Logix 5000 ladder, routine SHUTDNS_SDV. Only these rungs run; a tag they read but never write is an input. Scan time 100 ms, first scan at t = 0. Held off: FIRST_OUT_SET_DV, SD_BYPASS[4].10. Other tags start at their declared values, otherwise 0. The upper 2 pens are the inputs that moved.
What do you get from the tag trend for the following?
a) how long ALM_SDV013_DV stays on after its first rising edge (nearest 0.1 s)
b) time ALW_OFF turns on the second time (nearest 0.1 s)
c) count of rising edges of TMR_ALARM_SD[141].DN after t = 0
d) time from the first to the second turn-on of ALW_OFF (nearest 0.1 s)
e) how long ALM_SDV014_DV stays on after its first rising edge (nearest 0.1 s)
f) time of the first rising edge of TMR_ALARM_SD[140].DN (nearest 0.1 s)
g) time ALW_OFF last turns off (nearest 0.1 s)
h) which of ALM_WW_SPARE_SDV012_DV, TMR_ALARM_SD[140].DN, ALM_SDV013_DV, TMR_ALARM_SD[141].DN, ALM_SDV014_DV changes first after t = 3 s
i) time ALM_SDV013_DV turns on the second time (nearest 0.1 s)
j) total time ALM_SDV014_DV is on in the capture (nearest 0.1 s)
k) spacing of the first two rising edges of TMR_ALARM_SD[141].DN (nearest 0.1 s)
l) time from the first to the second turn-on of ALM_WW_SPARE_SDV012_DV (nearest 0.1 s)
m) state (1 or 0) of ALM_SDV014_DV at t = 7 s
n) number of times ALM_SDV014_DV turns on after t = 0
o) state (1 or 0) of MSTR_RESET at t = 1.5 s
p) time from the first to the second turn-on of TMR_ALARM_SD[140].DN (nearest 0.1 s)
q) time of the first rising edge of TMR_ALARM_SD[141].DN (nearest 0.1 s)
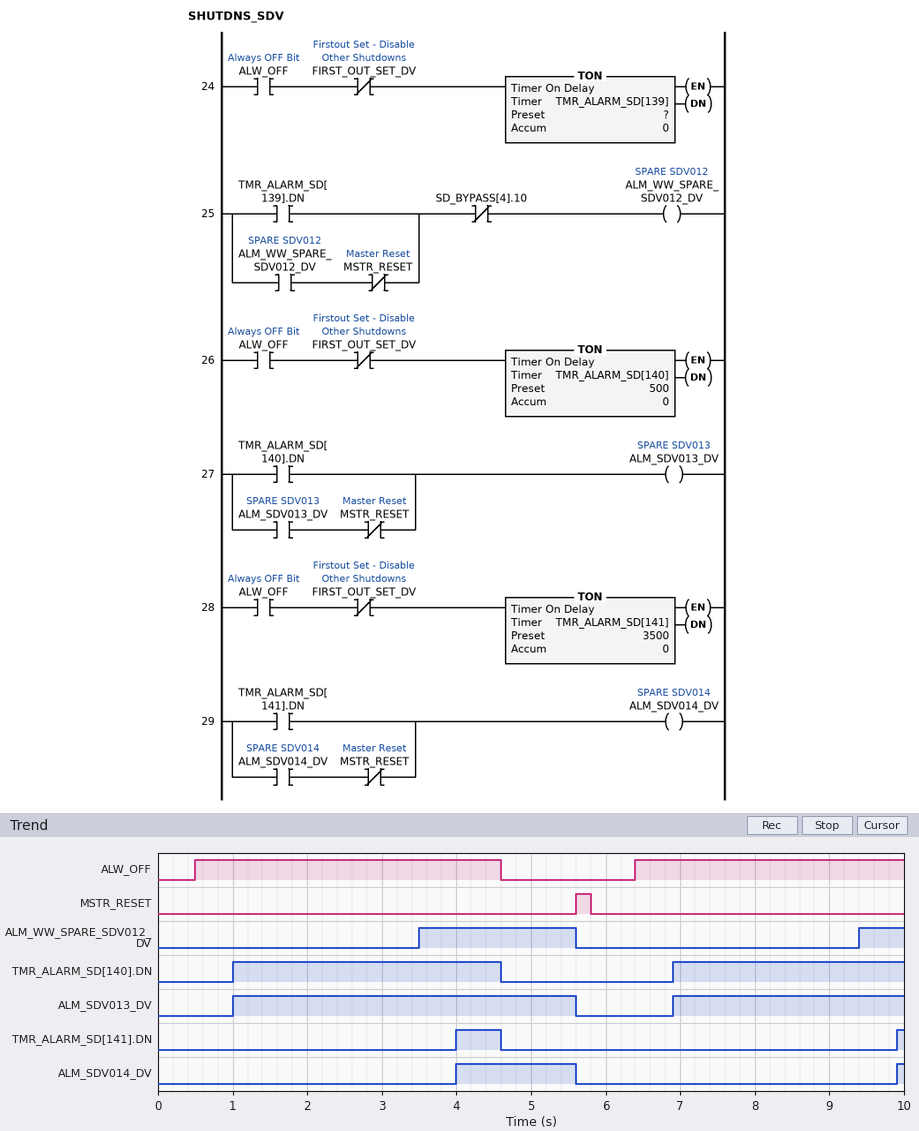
4.6 s
6.4 s
2
5.9 s
1.6 s
1.0 s
4.6 s
ALM_WW_SPARE_SDV012_DV
6.9 s
1.7 s
5.9 s
5.9 s
0
2
0
5.9 s
4.0 s
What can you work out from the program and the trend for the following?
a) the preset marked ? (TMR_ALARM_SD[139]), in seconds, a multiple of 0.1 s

3.0 s
